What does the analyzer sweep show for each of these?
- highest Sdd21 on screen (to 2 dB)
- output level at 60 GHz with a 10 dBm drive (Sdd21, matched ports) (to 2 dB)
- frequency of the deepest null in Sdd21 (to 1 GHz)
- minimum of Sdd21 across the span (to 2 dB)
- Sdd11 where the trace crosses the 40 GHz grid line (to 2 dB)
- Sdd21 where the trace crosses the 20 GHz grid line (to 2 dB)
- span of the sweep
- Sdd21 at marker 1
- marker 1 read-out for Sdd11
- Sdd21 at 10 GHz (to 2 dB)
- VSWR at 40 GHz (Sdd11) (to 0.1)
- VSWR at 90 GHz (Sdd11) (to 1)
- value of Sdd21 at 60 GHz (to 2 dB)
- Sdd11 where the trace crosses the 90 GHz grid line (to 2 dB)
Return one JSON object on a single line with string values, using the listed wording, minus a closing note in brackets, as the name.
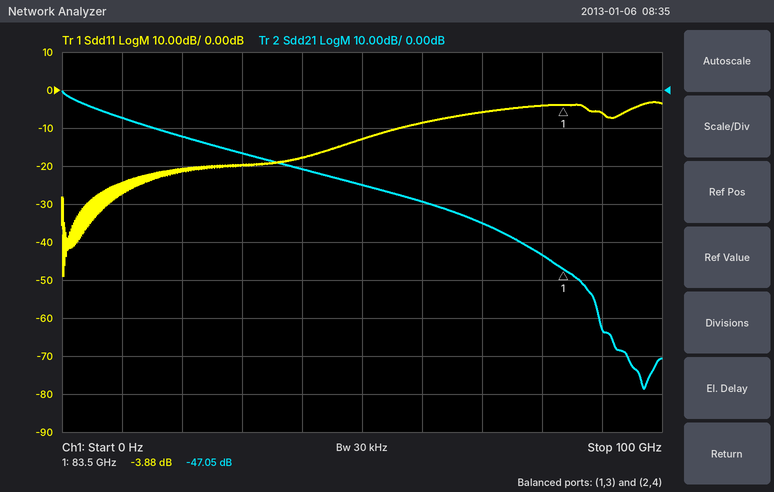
{"highest Sdd21 on screen": "0 dB", "output level at 60 GHz with a 10 dBm drive (Sdd21, matched ports)": "-20 dBm", "frequency of the deepest null in Sdd21": "97 GHz", "minimum of Sdd21 across the span": "-78 dB", "Sdd11 where the trace crosses the 40 GHz grid line": "-18 dB", "Sdd21 where the trace crosses the 20 GHz grid line": "-12 dB", "span of the sweep": "100 GHz", "Sdd21 at marker 1": "-47.05 dB", "marker 1 read-out for Sdd11": "-3.88 dB", "Sdd21 at 10 GHz": "-8 dB", "VSWR at 40 GHz (Sdd11)": "1.3", "VSWR at 90 GHz (Sdd11)": "3", "value of Sdd21 at 60 GHz": "-30 dB", "Sdd11 where the trace crosses the 90 GHz grid line": "-6 dB"}
